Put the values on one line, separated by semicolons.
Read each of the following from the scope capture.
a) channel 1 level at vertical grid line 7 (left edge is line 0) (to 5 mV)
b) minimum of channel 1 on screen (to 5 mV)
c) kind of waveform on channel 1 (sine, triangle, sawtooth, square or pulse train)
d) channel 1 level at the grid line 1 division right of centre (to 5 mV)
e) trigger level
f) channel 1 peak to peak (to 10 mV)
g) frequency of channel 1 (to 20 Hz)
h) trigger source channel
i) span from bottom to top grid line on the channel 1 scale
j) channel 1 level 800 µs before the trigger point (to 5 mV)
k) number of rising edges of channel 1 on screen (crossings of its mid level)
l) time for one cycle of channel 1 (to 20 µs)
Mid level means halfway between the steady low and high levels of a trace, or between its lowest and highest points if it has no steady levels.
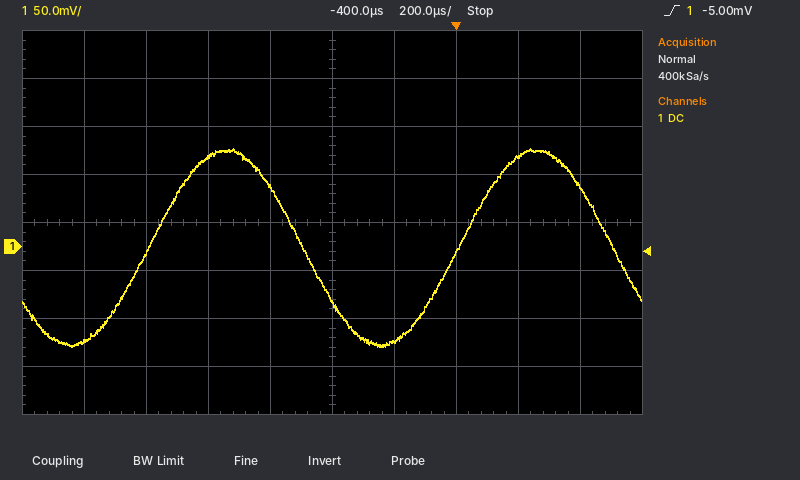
-5 mV; -105 mV; sine; -100 mV; -5.00 mV; 210 mV; 1.00 kHz; channel 1; 400 mV; 95 mV; 2; 1.00 ms
